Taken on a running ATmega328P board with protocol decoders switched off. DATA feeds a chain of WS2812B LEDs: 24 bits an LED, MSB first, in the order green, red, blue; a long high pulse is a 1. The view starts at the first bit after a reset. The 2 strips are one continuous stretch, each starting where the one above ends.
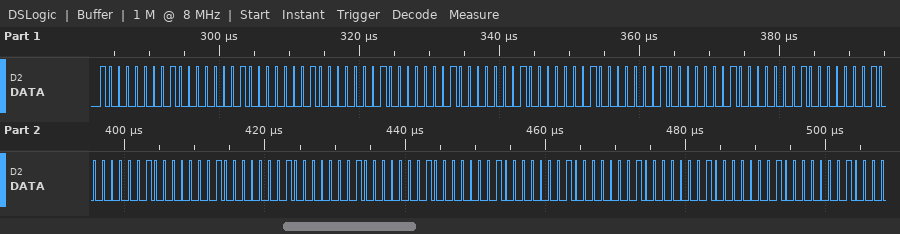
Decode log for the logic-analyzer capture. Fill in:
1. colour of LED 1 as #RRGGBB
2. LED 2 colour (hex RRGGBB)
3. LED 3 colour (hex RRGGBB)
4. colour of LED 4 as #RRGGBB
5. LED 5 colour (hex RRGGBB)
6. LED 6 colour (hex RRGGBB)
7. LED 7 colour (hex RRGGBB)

#808080
#808080
#808080
#808080
#808080
#808080
#808080
